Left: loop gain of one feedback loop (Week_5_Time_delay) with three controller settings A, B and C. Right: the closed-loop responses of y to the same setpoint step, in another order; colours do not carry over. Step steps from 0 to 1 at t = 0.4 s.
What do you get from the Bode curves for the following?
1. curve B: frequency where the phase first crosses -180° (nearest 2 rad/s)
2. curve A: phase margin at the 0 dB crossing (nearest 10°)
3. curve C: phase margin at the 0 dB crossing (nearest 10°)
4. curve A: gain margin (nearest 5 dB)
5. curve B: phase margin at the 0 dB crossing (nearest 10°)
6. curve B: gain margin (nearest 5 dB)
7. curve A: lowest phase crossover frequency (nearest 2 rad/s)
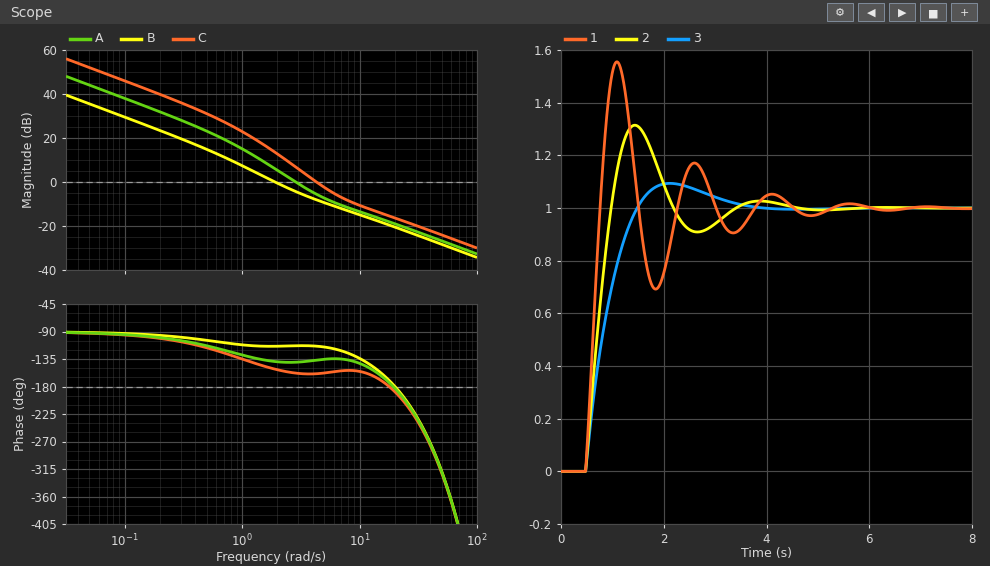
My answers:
20 rad/s
40°
20°
20 dB
70°
20 dB
20 rad/s
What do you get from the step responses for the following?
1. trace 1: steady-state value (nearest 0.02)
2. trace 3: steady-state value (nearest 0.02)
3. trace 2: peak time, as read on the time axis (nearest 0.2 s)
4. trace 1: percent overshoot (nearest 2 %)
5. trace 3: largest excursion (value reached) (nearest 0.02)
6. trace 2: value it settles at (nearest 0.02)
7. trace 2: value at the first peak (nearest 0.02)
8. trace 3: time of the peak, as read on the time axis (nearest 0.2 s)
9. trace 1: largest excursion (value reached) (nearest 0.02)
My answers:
1.00
1.00
1.4 s
56 %
1.10
1.00
1.32
2.2 s
1.56
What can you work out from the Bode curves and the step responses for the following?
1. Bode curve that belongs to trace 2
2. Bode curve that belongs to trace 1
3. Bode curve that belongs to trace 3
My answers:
A
C
B
